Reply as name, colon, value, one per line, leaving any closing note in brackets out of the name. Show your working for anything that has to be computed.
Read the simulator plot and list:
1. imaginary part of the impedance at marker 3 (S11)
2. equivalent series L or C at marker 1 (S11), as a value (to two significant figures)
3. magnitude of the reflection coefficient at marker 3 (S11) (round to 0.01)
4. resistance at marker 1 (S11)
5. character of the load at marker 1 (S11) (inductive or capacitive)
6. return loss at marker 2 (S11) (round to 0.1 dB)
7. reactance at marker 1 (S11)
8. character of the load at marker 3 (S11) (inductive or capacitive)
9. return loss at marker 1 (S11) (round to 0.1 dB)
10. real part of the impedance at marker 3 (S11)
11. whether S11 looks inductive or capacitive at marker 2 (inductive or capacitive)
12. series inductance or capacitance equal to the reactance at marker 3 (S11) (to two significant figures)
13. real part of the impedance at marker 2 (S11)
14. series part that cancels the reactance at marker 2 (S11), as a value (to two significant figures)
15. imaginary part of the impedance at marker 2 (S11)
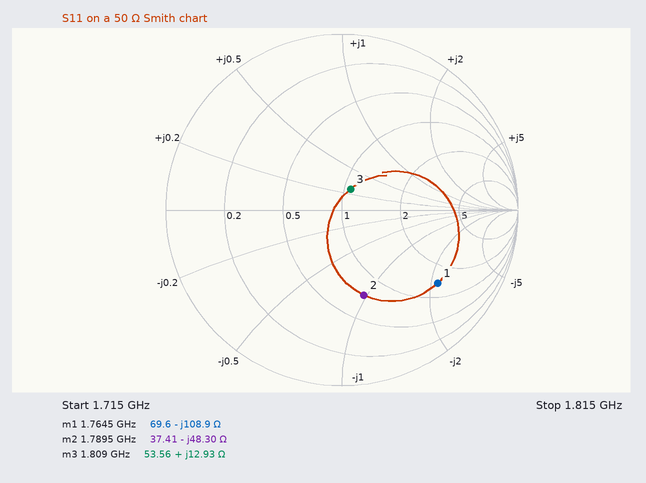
imaginary part of the impedance at marker 3: +12.93 Ω
equivalent series L or C at marker 1 (S11), as a value: C = 1/(2π × 1.7645 GHz × 108.9 Ω) ≈ 828 fF, so 830 fF to two significant figures
magnitude of the reflection coefficient at marker 3 (S11): 0.13
resistance at marker 1: 69.6 Ω
character of the load at marker 1 (S11): capacitive
return loss at marker 2 (S11): 6.0 dB
reactance at marker 1: -108.9 Ω
character of the load at marker 3 (S11): inductive
return loss at marker 1 (S11): 3.3 dB
real part of the impedance at marker 3: 53.56 Ω
whether S11 looks inductive or capacitive at marker 2: capacitive
series inductance or capacitance equal to the reactance at marker 3 (S11): L = 12.93 Ω/(2π × 1.809 GHz) ≈ 1.1 nH
real part of the impedance at marker 2: 37.41 Ω
series part that cancels the reactance at marker 2 (S11), as a value: L = 48.3 Ω/(2π × 1.7895 GHz) ≈ 4.3 nH
imaginary part of the impedance at marker 2: -48.30 Ω
